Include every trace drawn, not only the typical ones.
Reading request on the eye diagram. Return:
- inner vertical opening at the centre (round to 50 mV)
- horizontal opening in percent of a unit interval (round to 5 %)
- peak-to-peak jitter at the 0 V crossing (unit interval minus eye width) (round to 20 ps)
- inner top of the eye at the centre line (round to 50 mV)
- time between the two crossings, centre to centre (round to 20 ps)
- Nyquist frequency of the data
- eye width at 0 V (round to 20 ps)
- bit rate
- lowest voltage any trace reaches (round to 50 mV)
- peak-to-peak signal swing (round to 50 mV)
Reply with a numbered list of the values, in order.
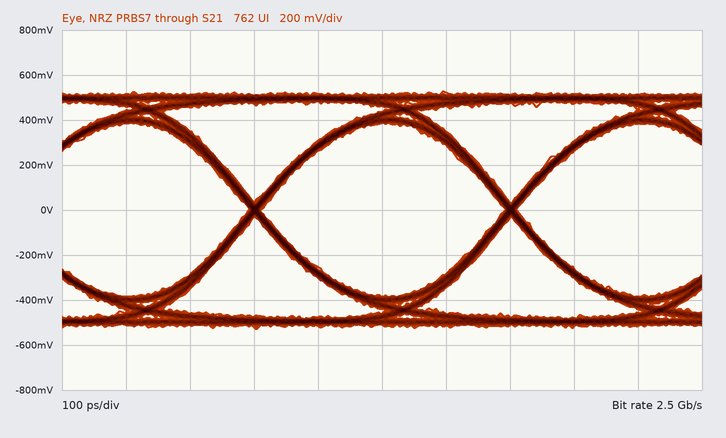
1. 750 mV
2. 95 %
3. 20 ps
4. 400 mV
5. 400 ps
6. 1.25 GHz
7. 380 ps
8. 2.5 Gb/s
9. -550 mV
10. 1.05 V
